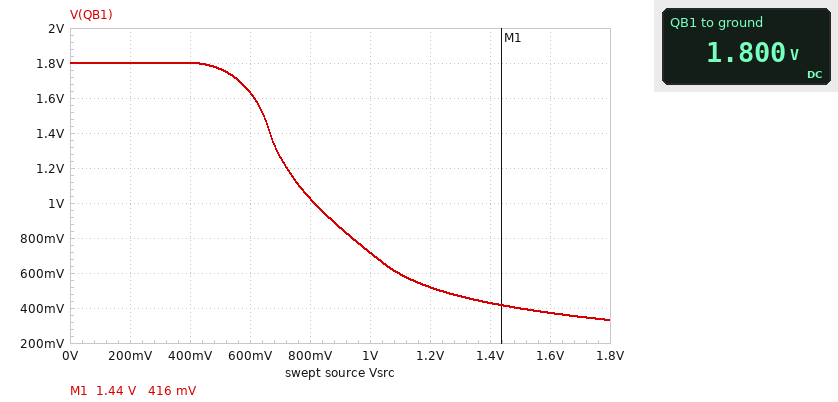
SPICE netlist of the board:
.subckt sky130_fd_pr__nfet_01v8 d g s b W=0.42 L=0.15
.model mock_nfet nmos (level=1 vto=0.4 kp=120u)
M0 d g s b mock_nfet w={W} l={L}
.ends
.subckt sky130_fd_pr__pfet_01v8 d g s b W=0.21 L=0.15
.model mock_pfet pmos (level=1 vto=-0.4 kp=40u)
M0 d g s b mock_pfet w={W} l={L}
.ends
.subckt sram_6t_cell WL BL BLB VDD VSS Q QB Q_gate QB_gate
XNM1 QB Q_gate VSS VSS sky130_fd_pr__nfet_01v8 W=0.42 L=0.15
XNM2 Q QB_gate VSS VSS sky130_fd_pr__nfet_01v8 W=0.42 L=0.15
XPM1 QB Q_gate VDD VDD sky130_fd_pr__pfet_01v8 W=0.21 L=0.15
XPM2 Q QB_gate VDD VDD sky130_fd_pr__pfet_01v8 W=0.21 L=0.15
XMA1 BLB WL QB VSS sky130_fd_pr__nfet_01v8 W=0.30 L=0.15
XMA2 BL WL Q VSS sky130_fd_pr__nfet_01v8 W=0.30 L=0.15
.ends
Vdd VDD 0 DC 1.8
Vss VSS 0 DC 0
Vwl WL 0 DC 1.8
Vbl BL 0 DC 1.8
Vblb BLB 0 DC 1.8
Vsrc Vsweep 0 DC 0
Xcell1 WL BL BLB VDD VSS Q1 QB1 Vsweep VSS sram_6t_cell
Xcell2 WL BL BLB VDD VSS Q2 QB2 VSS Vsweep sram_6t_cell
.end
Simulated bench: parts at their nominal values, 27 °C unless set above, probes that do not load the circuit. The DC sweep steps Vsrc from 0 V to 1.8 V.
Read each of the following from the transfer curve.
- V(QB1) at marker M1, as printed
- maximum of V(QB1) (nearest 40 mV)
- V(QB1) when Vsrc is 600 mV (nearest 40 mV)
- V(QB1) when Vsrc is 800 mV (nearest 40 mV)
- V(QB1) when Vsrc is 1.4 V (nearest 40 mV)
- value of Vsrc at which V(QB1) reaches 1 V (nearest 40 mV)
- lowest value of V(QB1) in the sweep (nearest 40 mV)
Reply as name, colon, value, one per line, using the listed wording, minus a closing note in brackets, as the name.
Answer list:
V(QB1) at marker M1, as printed: 416 mV
maximum of V(QB1): 1.80 V
V(QB1) when Vsrc is 600 mV: 1.64 V
V(QB1) when Vsrc is 800 mV: 1.04 V
V(QB1) when Vsrc is 1.4 V: 440 mV
value of Vsrc at which V(QB1) reaches 1 V: 800 mV
lowest value of V(QB1) in the sweep: 320 mV
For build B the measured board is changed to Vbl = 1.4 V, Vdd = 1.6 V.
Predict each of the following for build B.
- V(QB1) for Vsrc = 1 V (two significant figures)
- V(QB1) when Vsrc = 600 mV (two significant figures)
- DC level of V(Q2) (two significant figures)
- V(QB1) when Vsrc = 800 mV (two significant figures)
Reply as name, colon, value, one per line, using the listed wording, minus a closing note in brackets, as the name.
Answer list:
V(QB1) for Vsrc = 1 V: 700 mV
V(QB1) when Vsrc = 600 mV: 1.4 V
DC level of V(Q2): 1.6 V
V(QB1) when Vsrc = 800 mV: 970 mV
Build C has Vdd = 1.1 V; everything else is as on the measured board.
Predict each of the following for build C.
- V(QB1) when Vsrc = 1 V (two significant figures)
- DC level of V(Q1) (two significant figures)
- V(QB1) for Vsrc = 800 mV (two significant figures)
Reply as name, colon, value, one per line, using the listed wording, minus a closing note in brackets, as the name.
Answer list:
V(QB1) when Vsrc = 1 V: 690 mV
DC level of V(Q1): 1.2 V
V(QB1) for Vsrc = 800 mV: 930 mV
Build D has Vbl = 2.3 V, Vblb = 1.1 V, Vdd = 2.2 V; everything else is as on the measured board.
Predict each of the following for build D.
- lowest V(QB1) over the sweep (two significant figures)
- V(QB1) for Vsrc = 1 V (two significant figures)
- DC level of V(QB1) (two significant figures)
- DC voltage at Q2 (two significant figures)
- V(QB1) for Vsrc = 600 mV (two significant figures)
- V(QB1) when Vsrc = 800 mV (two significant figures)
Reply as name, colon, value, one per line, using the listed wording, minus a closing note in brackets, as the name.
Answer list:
lowest V(QB1) over the sweep: 310 mV
V(QB1) for Vsrc = 1 V: 730 mV
DC level of V(QB1): 2.1 V
DC voltage at Q2: 2.2 V
V(QB1) for Vsrc = 600 mV: 1.9 V
V(QB1) when Vsrc = 800 mV: 1.1 V
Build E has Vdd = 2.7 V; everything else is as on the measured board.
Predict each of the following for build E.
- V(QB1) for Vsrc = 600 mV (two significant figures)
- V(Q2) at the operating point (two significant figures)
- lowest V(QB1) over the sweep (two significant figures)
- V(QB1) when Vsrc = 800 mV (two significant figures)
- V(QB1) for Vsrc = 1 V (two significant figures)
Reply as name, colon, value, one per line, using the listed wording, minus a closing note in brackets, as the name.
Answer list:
V(QB1) for Vsrc = 600 mV: 2.6 V
V(Q2) at the operating point: 2.7 V
lowest V(QB1) over the sweep: 340 mV
V(QB1) when Vsrc = 800 mV: 2.3 V
V(QB1) for Vsrc = 1 V: 1.1 V
